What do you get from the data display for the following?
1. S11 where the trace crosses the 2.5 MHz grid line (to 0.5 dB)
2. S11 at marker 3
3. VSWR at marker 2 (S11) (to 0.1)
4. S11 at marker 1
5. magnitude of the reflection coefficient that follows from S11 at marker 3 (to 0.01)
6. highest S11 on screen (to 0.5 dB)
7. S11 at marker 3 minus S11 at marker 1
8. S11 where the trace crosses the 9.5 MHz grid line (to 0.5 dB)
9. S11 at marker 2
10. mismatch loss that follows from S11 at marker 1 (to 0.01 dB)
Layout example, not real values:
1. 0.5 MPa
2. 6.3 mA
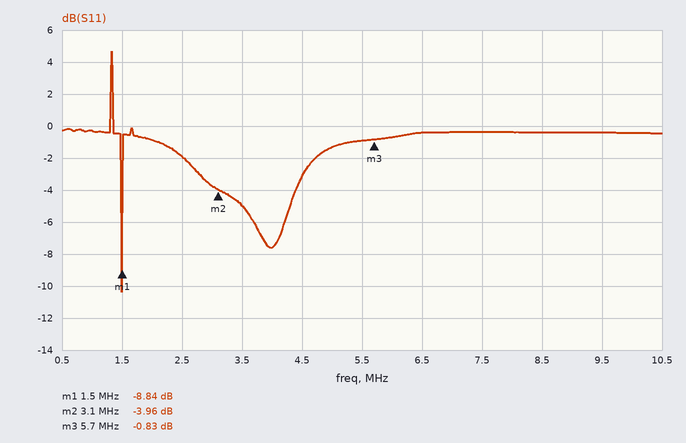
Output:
1. -2.0 dB
2. -0.83 dB
3. 4.5
4. -8.84 dB
5. 0.91
6. 4.5 dB
7. 8.01 dB
8. -0.5 dB
9. -3.96 dB
10. 0.61 dB
